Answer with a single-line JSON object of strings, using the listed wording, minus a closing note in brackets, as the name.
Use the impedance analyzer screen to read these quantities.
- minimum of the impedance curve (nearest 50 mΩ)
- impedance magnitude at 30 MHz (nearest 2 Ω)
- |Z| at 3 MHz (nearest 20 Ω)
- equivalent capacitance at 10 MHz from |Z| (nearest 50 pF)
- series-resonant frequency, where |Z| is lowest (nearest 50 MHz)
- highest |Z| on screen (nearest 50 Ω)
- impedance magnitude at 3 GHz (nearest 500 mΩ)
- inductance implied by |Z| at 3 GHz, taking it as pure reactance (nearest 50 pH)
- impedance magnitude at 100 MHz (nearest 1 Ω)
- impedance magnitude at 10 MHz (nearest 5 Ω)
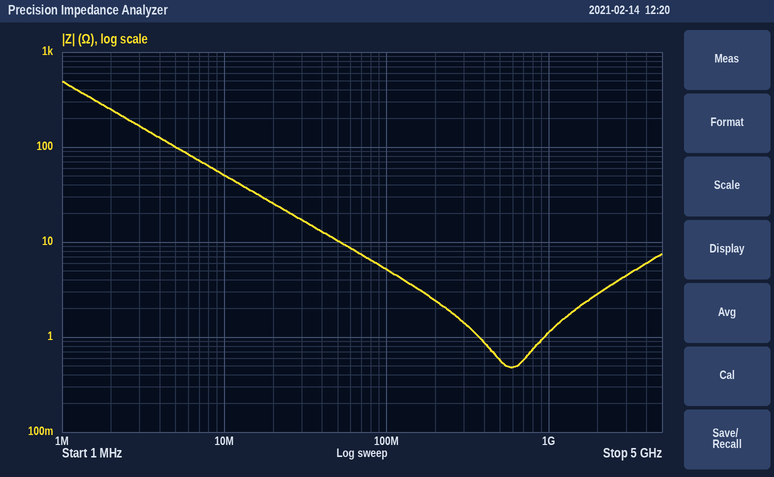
{"minimum of the impedance curve": "500 mΩ", "impedance magnitude at 30 MHz": "18 Ω", "|Z| at 3 MHz": "160 Ω", "equivalent capacitance at 10 MHz from |Z|": "300 pF", "series-resonant frequency, where |Z| is lowest": "600 MHz", "highest |Z| on screen": "500 Ω", "impedance magnitude at 3 GHz": "4.5 Ω", "inductance implied by |Z| at 3 GHz, taking it as pure reactance": "250 pH", "impedance magnitude at 100 MHz": "5 Ω", "impedance magnitude at 10 MHz": "50 Ω"}
